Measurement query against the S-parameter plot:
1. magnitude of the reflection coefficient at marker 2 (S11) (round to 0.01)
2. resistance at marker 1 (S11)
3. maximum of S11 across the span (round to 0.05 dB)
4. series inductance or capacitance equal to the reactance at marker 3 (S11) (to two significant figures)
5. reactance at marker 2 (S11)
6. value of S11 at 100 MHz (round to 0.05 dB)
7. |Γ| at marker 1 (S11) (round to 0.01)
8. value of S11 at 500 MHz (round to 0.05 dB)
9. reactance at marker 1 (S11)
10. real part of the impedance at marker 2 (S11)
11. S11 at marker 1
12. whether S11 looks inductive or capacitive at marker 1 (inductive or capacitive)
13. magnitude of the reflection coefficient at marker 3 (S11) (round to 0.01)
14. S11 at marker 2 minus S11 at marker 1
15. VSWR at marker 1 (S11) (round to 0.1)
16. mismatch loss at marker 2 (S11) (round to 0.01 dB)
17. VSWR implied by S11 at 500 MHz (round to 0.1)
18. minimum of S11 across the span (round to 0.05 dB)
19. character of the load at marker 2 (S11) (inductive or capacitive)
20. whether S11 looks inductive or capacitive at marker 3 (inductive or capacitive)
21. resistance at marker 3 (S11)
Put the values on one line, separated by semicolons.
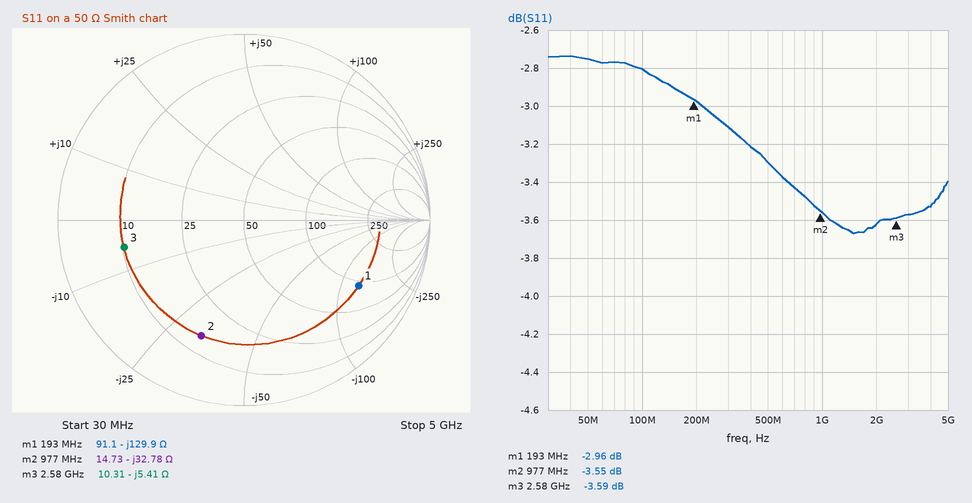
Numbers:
0.66; 91.1 Ω; -2.75 dB; 11 pF; -32.78 Ω; -2.80 dB; 0.71; -3.30 dB; -129.9 Ω; 14.73 Ω; -2.96 dB; capacitive; 0.66; -0.59 dB; 5.9; 2.53 dB; 5.3; -3.65 dB; capacitive; capacitive; 10.31 Ω
